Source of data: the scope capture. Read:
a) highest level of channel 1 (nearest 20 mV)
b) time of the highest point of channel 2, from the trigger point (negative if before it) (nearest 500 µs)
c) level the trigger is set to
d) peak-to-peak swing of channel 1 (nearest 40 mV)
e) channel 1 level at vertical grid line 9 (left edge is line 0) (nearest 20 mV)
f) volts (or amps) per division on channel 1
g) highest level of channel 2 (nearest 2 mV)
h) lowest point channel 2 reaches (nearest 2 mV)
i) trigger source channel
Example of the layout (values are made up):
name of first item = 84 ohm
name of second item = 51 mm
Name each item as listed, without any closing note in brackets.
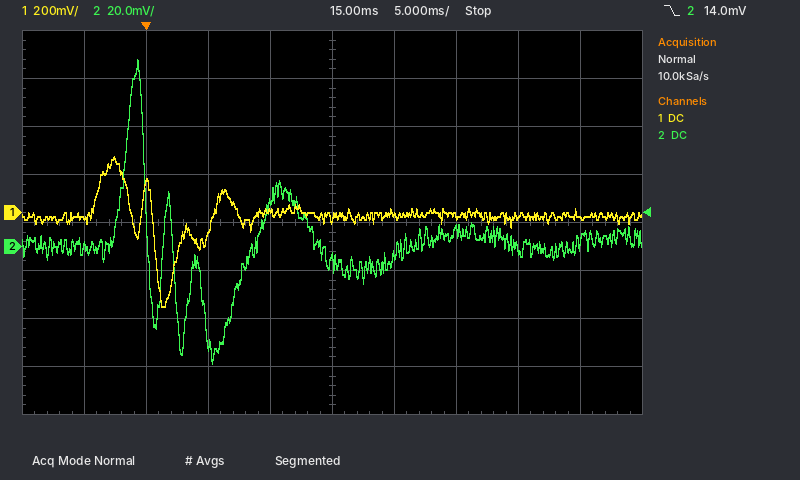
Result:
highest level of channel 1 = 240 mV
time of the highest point of channel 2, from the trigger point (negative if before it) = -500 µs
level the trigger is set to = 14.0 mV
peak-to-peak swing of channel 1 = 640 mV
channel 1 level at vertical grid line 9 (left edge is line 0) = -20 mV
volts (or amps) per division on channel 1 = 200 mV
highest level of channel 2 = 78 mV
lowest point channel 2 reaches = -48 mV
trigger source channel = channel 2
